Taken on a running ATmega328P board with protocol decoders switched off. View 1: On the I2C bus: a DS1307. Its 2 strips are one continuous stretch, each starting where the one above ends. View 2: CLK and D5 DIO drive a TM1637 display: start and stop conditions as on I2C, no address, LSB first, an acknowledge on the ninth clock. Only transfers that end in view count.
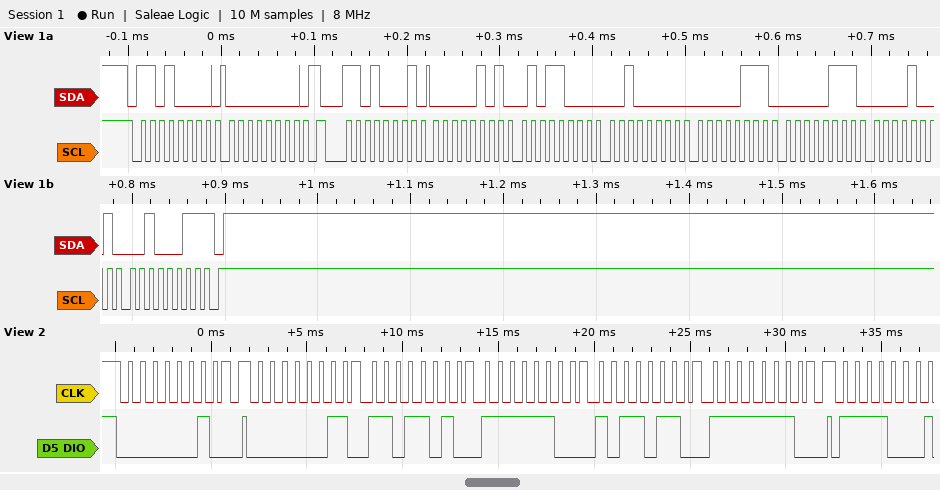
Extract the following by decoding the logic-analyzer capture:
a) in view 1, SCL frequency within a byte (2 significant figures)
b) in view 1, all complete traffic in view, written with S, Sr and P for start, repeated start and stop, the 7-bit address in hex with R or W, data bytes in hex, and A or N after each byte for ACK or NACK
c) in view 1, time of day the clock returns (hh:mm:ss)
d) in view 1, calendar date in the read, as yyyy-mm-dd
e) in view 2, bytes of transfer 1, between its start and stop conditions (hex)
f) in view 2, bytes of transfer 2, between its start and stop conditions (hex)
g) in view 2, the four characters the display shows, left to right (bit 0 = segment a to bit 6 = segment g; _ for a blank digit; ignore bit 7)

100 kHz
S 68W A 00 A Sr 68R A 05 A 58 A 20 A 07 A 07 A 09 A 23 N P
20:58:05
2023-09-07
40
C0 5B 3F 6D 7F
2058
